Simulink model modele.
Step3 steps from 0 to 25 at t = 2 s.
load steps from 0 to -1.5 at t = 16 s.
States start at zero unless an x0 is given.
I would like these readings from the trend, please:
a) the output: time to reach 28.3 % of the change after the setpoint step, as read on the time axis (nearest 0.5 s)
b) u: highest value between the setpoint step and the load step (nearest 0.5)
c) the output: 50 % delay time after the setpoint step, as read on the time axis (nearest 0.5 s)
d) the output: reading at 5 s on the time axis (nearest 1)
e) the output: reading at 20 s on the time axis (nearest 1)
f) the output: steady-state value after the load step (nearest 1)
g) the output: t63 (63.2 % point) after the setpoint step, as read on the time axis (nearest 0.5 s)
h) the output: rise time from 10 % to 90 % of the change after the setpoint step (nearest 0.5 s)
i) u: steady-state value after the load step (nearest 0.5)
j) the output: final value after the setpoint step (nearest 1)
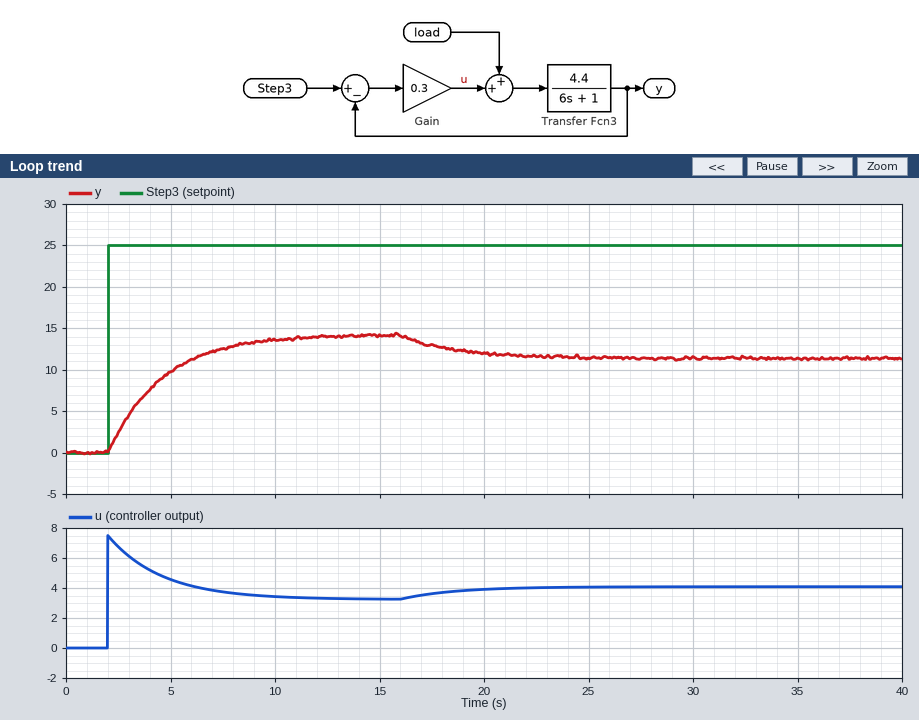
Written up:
3.0 s
7.5
4.0 s
10
12
11
4.5 s
5.5 s
4.0
14
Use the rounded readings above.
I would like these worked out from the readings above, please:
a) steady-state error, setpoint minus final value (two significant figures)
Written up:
11
